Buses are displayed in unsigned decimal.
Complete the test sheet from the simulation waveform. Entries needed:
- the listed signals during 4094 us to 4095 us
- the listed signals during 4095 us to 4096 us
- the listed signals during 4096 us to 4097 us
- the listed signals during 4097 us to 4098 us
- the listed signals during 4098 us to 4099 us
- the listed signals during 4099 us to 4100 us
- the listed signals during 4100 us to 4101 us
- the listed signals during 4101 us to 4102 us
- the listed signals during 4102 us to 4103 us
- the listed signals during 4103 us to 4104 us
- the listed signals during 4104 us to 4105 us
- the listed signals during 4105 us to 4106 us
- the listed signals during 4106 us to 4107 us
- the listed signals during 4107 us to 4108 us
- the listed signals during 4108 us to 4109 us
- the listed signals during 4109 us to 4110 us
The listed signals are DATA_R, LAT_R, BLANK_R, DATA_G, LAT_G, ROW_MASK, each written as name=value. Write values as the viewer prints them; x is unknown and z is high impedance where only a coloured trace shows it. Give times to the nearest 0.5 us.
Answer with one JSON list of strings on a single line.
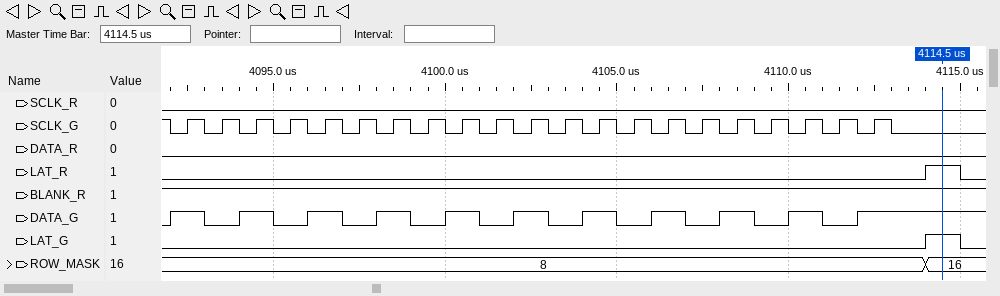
["DATA_R=0, LAT_R=0, BLANK_R=1, DATA_G=1, LAT_G=0, ROW_MASK=8", "DATA_R=0, LAT_R=0, BLANK_R=1, DATA_G=0, LAT_G=0, ROW_MASK=8", "DATA_R=0, LAT_R=0, BLANK_R=1, DATA_G=1, LAT_G=0, ROW_MASK=8", "DATA_R=0, LAT_R=0, BLANK_R=1, DATA_G=0, LAT_G=0, ROW_MASK=8", "DATA_R=0, LAT_R=0, BLANK_R=1, DATA_G=1, LAT_G=0, ROW_MASK=8", "DATA_R=0, LAT_R=0, BLANK_R=1, DATA_G=0, LAT_G=0, ROW_MASK=8", "DATA_R=0, LAT_R=0, BLANK_R=1, DATA_G=1, LAT_G=0, ROW_MASK=8", "DATA_R=0, LAT_R=0, BLANK_R=1, DATA_G=0, LAT_G=0, ROW_MASK=8", "DATA_R=0, LAT_R=0, BLANK_R=1, DATA_G=1, LAT_G=0, ROW_MASK=8", "DATA_R=0, LAT_R=0, BLANK_R=1, DATA_G=0, LAT_G=0, ROW_MASK=8", "DATA_R=0, LAT_R=0, BLANK_R=1, DATA_G=1, LAT_G=0, ROW_MASK=8", "DATA_R=0, LAT_R=0, BLANK_R=1, DATA_G=0, LAT_G=0, ROW_MASK=8", "DATA_R=0, LAT_R=0, BLANK_R=1, DATA_G=1, LAT_G=0, ROW_MASK=8", "DATA_R=0, LAT_R=0, BLANK_R=1, DATA_G=0, LAT_G=0, ROW_MASK=8", "DATA_R=0, LAT_R=0, BLANK_R=1, DATA_G=1, LAT_G=0, ROW_MASK=8", "DATA_R=0, LAT_R=0, BLANK_R=1, DATA_G=0, LAT_G=0, ROW_MASK=8"]
